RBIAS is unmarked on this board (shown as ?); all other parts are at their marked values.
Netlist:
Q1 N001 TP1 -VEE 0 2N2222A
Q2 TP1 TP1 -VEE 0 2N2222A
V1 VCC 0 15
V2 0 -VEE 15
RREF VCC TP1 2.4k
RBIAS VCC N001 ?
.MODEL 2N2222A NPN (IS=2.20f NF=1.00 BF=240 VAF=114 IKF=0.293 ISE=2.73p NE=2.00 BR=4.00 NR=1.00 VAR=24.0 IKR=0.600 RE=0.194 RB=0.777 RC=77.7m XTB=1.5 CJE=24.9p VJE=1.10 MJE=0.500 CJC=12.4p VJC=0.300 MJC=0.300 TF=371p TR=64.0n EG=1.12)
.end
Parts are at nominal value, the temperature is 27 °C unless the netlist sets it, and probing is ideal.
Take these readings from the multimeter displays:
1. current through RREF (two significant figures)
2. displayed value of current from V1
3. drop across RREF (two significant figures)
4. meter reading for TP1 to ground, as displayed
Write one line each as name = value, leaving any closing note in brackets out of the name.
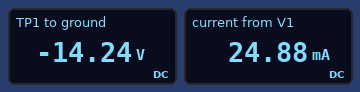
current through RREF = 12 mA
displayed value of current from V1 = 24.88 mA
drop across RREF = 29 V
meter reading for TP1 to ground, as displayed = -14.24 V
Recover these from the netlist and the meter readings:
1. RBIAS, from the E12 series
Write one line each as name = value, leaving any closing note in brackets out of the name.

RBIAS, from the E12 series = 1.8 kΩ
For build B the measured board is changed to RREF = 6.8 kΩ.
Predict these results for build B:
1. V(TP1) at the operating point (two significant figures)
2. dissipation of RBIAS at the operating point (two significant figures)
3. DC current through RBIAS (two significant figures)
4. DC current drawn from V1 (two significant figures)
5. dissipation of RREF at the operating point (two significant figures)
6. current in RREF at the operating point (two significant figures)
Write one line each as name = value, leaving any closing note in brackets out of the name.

V(TP1) at the operating point = -14 V
dissipation of RBIAS at the operating point = 45 mW
DC current through RBIAS = 5.0 mA
DC current drawn from V1 = 9.3 mA
dissipation of RREF at the operating point = 130 mW
current in RREF at the operating point = 4.3 mA
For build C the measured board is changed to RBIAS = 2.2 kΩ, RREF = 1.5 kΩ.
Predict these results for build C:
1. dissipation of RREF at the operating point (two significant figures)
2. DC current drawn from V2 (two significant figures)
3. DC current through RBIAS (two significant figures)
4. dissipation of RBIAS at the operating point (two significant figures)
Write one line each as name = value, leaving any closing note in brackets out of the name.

dissipation of RREF at the operating point = 570 mW
DC current drawn from V2 = 33 mA
DC current through RBIAS = 14 mA
dissipation of RBIAS at the operating point = 410 mW
